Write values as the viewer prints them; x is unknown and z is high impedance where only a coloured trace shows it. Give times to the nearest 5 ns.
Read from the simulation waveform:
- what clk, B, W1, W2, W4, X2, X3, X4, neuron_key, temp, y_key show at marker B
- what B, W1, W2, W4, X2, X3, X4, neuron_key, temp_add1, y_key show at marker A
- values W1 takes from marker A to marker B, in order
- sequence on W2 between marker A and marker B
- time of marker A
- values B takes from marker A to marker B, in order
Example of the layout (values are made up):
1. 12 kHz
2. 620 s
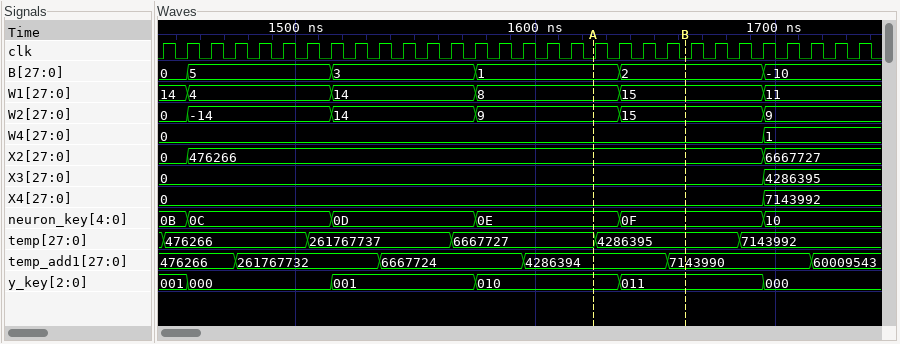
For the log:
1. clk=0, B=2, W1=15, W2=15, W4=0, X2=476266, X3=0, X4=0, neuron_key=0F, temp=4286395, y_key=011
2. B=1, W1=8, W2=9, W4=0, X2=476266, X3=0, X4=0, neuron_key=0E, temp_add1=4286394, y_key=010
3. 8, 15
4. 9, 15
5. 1625 ns
6. 1, 2
